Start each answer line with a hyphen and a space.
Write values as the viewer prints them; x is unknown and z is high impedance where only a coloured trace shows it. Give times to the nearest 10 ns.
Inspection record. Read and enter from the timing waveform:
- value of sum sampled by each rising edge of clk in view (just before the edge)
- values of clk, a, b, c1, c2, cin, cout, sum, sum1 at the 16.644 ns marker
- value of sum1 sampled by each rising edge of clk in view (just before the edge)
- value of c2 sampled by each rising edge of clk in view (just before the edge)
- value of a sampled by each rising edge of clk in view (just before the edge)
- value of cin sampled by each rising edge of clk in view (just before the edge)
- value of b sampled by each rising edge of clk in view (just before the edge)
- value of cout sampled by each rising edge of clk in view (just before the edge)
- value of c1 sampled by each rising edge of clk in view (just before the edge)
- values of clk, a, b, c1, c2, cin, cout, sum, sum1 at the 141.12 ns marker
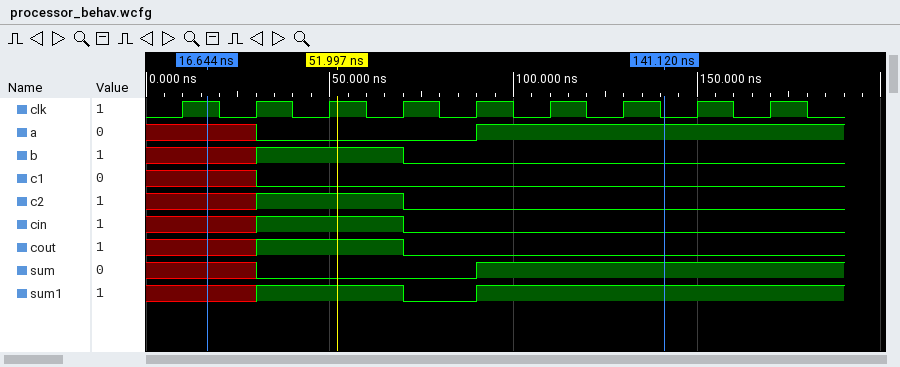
- x x 0 0 0 1 1 1 1
- clk=1, a=x, b=x, c1=x, c2=x, cin=x, cout=x, sum=x, sum1=x
- x x 1 1 0 1 1 1 1
- x x 1 1 0 0 0 0 0
- x x 0 0 0 1 1 1 1
- x x 1 1 0 0 0 0 0
- x x 1 1 0 0 0 0 0
- x x 1 1 0 0 0 0 0
- x x 0 0 0 0 0 0 0
- clk=0, a=1, b=0, c1=0, c2=0, cin=0, cout=0, sum=1, sum1=1
